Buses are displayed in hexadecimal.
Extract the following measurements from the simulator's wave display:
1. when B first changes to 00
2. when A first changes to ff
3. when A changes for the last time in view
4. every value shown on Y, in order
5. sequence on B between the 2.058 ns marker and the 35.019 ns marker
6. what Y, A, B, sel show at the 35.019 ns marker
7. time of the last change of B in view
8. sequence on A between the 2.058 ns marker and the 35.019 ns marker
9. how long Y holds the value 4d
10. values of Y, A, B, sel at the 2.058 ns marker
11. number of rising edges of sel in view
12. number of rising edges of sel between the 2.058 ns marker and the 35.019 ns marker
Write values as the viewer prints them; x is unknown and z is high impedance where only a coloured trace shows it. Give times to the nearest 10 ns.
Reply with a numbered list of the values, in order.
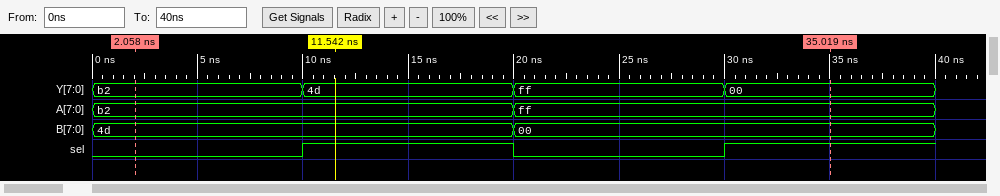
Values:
1. 20 ns
2. 20 ns
3. 20 ns
4. b2, 4d, ff, 00
5. 4d, 00
6. Y=00, A=ff, B=00, sel=1
7. 20 ns
8. b2, ff
9. 10 ns
10. Y=b2, A=b2, B=4d, sel=0
11. 2
12. 2
